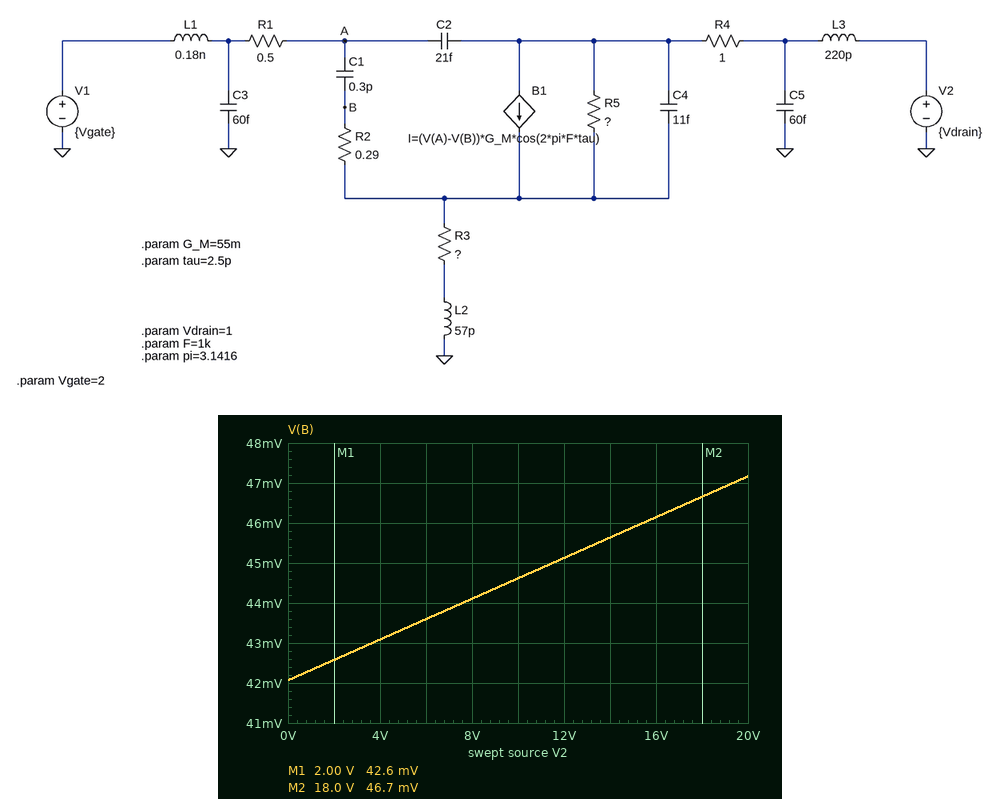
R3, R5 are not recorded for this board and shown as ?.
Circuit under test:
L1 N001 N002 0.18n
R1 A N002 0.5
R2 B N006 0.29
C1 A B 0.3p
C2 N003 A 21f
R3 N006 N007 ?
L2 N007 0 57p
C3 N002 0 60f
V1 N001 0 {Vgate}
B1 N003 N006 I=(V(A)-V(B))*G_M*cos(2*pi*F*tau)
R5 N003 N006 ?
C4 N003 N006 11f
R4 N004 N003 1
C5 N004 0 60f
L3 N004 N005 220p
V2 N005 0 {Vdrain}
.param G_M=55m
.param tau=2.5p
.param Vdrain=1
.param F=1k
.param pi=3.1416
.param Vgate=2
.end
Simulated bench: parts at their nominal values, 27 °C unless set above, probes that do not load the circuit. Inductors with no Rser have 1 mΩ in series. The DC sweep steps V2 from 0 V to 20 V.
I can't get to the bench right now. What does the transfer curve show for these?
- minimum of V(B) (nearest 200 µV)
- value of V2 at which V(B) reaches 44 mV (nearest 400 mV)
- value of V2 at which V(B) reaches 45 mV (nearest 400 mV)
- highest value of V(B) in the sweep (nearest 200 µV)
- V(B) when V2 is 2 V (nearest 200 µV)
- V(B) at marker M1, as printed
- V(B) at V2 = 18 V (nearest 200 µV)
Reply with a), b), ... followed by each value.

a) 42.0 mV
b) 7.6 V
c) 11.6 V
d) 47.2 mV
e) 42.6 mV
f) 42.6 mV
g) 46.6 mV
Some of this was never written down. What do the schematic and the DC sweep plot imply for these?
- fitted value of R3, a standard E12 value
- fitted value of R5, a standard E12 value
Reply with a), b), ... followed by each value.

a) 0.39 Ω
b) 1.5 kΩ
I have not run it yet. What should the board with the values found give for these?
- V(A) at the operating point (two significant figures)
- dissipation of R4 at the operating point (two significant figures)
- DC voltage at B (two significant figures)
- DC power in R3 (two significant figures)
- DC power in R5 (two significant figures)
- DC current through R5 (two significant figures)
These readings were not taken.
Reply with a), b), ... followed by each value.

a) 2.0 V
b) 12 mW
c) 42 mV
d) 4.6 mW
e) 480 µW
f) 570 µA
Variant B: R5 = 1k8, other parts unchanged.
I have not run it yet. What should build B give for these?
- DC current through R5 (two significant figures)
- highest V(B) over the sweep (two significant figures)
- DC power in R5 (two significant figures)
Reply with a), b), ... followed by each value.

a) 470 µA
b) 46 mV
c) 400 µW
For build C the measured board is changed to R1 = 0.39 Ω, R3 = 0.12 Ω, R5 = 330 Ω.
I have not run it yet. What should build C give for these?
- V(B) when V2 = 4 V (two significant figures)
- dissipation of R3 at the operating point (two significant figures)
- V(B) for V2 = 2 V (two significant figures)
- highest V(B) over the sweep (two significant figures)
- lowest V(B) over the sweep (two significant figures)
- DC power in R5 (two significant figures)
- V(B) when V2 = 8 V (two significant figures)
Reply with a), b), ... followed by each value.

a) 15 mV
b) 1.5 mW
c) 14 mV
d) 20 mV
e) 13 mV
f) 2.3 mW
g) 16 mV
